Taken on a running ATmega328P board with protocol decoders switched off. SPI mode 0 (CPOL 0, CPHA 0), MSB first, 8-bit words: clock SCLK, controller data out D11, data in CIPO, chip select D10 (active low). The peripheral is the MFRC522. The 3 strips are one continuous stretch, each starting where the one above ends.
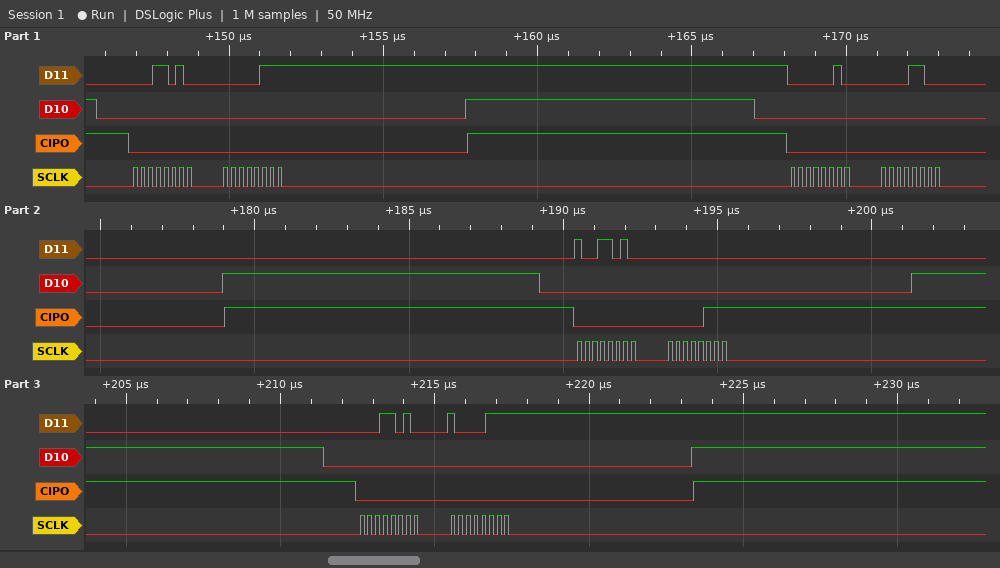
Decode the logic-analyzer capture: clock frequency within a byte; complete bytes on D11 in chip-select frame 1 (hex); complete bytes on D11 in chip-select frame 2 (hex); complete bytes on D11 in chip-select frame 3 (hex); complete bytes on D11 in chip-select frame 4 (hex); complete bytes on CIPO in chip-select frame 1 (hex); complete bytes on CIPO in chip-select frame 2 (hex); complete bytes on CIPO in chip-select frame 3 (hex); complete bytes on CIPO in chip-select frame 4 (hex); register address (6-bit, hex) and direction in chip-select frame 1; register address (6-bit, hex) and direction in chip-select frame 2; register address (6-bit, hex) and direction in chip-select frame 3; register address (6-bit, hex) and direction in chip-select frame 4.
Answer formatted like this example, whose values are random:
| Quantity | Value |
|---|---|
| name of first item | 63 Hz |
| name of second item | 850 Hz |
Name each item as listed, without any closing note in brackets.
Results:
| Quantity | Value |
|---|---|
| clock frequency within a byte | 4 MHz |
| complete bytes on D11 in chip-select frame 1 | 1A 07 |
| complete bytes on D11 in chip-select frame 2 | 02 0C |
| complete bytes on D11 in chip-select frame 3 | 9A 00 |
| complete bytes on D11 in chip-select frame 4 | 1A 87 |
| complete bytes on CIPO in chip-select frame 1 | 00 00 |
| complete bytes on CIPO in chip-select frame 2 | 00 00 |
| complete bytes on CIPO in chip-select frame 3 | 00 07 |
| complete bytes on CIPO in chip-select frame 4 | 00 00 |
| register address (6-bit, hex) and direction in chip-select frame 1 | 0x0D write |
| register address (6-bit, hex) and direction in chip-select frame 2 | 0x01 write |
| register address (6-bit, hex) and direction in chip-select frame 3 | 0x0D read |
| register address (6-bit, hex) and direction in chip-select frame 4 | 0x0D write |
